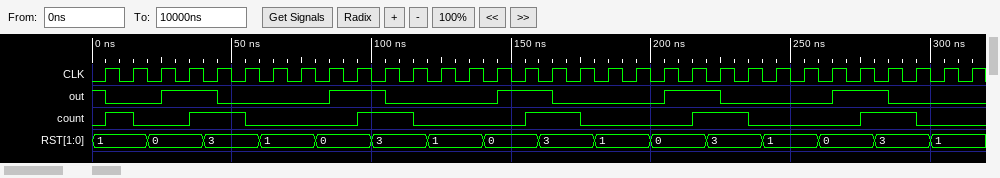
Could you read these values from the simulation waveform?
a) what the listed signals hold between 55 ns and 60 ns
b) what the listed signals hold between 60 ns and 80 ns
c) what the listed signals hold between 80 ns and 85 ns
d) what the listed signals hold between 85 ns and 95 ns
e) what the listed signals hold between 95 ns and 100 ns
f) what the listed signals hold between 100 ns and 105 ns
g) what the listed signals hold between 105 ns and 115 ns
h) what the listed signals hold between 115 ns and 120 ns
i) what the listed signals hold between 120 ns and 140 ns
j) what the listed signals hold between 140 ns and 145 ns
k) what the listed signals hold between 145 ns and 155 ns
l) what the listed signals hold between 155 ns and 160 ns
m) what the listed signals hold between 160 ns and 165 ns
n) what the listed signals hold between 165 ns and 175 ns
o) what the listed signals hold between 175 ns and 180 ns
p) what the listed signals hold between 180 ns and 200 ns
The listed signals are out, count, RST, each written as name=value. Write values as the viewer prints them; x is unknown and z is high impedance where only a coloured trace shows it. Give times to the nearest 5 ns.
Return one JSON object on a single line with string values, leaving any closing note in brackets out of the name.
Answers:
{"what the listed signals hold between 55 ns and 60 ns": "out=0, count=0, RST=3", "what the listed signals hold between 60 ns and 80 ns": "out=0, count=0, RST=1", "what the listed signals hold between 80 ns and 85 ns": "out=0, count=0, RST=0", "what the listed signals hold between 85 ns and 95 ns": "out=1, count=0, RST=0", "what the listed signals hold between 95 ns and 100 ns": "out=1, count=1, RST=0", "what the listed signals hold between 100 ns and 105 ns": "out=1, count=1, RST=3", "what the listed signals hold between 105 ns and 115 ns": "out=0, count=1, RST=3", "what the listed signals hold between 115 ns and 120 ns": "out=0, count=0, RST=3", "what the listed signals hold between 120 ns and 140 ns": "out=0, count=0, RST=1", "what the listed signals hold between 140 ns and 145 ns": "out=0, count=0, RST=0", "what the listed signals hold between 145 ns and 155 ns": "out=1, count=0, RST=0", "what the listed signals hold between 155 ns and 160 ns": "out=1, count=1, RST=0", "what the listed signals hold between 160 ns and 165 ns": "out=1, count=1, RST=3", "what the listed signals hold between 165 ns and 175 ns": "out=0, count=1, RST=3", "what the listed signals hold between 175 ns and 180 ns": "out=0, count=0, RST=3", "what the listed signals hold between 180 ns and 200 ns": "out=0, count=0, RST=1"}
